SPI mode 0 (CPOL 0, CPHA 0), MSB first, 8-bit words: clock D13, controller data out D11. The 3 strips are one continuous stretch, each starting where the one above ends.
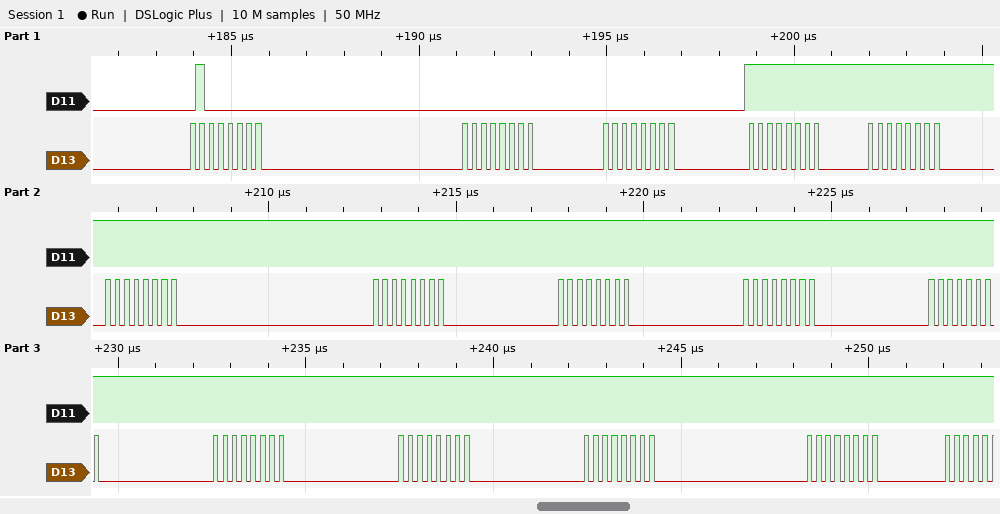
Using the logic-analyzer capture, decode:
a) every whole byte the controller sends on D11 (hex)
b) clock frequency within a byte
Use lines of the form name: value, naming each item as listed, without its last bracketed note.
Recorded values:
every whole byte the controller sends on D11: 40 00 00 FF FF FF FF FF FF FF FF FF FF FF
clock frequency within a byte: 4 MHz
